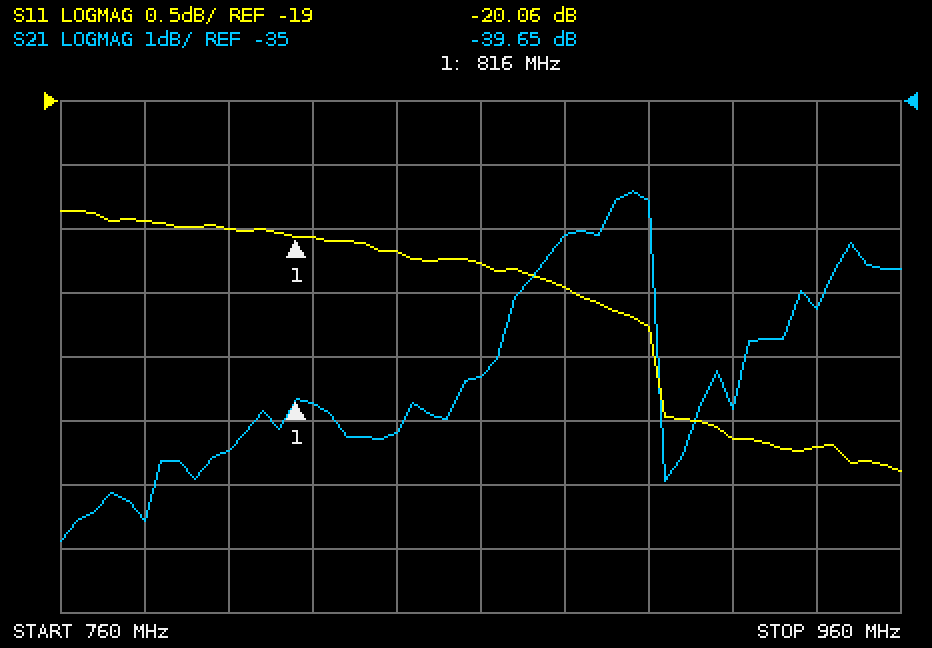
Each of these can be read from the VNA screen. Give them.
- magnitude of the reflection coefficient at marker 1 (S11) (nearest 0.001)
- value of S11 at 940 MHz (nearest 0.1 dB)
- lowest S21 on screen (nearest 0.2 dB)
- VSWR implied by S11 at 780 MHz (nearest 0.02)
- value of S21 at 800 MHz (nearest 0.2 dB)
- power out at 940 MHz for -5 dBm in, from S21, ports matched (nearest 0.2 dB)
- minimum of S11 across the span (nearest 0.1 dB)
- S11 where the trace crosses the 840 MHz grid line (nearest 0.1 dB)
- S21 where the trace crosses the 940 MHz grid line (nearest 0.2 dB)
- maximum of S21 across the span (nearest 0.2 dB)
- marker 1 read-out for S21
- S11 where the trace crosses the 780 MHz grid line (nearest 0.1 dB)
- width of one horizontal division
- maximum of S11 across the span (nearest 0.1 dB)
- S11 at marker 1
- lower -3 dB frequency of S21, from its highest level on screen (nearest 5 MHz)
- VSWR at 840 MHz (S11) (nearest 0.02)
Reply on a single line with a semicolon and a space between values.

0.099; -21.7 dB; -41.8 dB; 1.22; -40.4 dB; -43.2 dBm; -21.9 dB; -20.2 dB; -38.2 dB; -36.4 dB; -39.65 dB; -19.9 dB; 20 MHz; -19.9 dB; -20.06 dB; 855 MHz; 1.22
